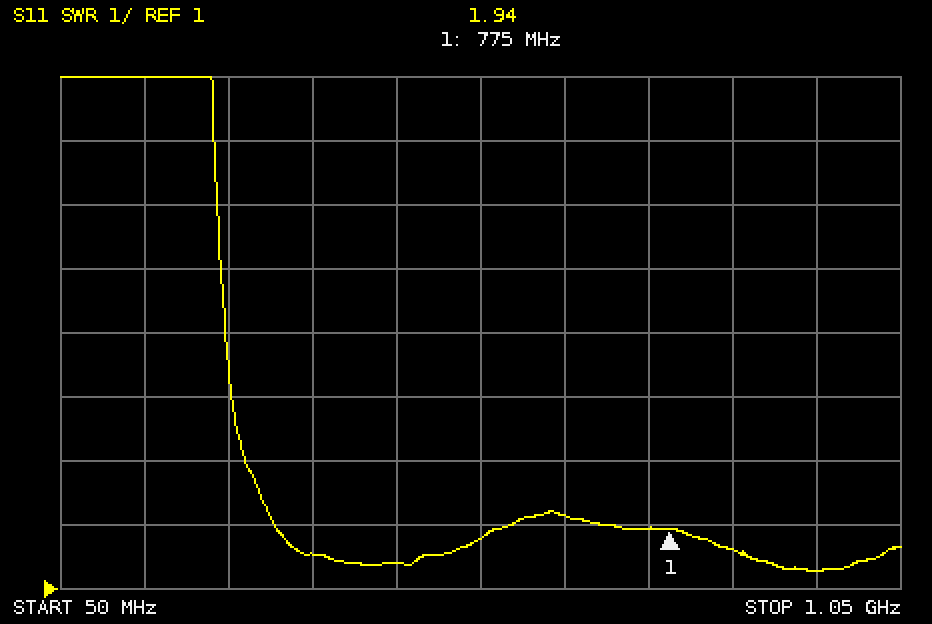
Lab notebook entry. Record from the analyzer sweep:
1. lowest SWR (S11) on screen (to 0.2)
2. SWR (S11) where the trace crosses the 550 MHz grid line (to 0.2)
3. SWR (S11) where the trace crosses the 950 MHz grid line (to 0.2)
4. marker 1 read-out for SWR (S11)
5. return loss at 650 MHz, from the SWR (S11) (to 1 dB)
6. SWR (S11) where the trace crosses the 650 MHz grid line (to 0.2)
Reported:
1.2
1.8
1.2
1.94
9 dB
2.2
